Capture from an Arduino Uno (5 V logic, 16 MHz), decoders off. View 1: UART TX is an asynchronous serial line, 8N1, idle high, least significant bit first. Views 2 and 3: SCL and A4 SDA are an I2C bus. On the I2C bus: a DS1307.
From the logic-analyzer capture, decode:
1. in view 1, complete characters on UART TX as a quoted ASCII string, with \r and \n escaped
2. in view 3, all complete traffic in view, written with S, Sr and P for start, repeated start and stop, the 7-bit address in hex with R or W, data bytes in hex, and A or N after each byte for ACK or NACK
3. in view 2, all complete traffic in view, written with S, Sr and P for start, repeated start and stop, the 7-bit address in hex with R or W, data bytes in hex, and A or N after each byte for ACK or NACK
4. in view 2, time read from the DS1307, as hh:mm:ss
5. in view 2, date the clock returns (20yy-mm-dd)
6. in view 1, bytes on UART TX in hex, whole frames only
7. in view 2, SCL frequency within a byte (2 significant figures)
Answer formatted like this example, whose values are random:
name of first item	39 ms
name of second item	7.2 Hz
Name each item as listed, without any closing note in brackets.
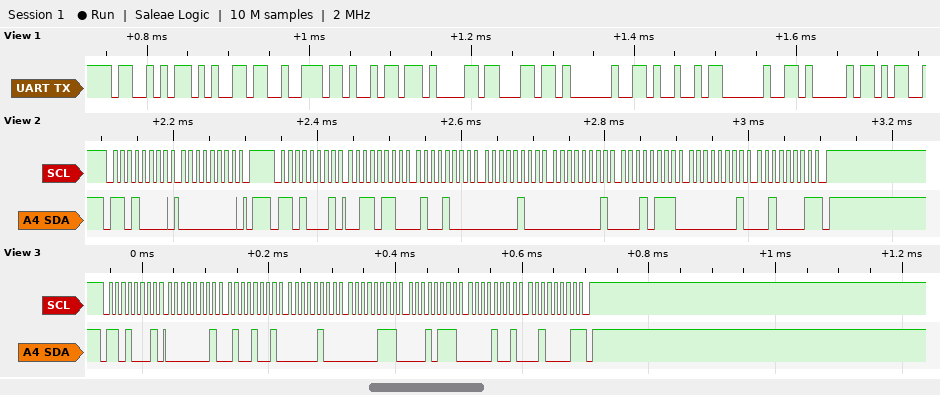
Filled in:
in view 1, complete characters on UART TX as a quoted ASCII string, with \r and \n escaped	"Serial I A"
in view 3, all complete traffic in view, written with S, Sr and P for start, repeated start and stop, the 7-bit address in hex with R or W, data bytes in hex, and A or N after each byte for ACK or NACK	S 68R A 01 A 49 A 04 A 07 A 17 A 09 A 21 N P
in view 2, all complete traffic in view, written with S, Sr and P for start, repeated start and stop, the 7-bit address in hex with R or W, data bytes in hex, and A or N after each byte for ACK or NACK	S 68W A 00 A P S 68R A 36 A 48 A 04 A 01 A 17 A 01 A 21 N P
in view 2, time read from the DS1307, as hh:mm:ss	04:48:36
in view 2, date the clock returns	2021-01-17
in view 1, bytes on UART TX in hex, whole frames only	53 65 72 69 61 6C 20 49 20 41
in view 2, SCL frequency within a byte	100 kHz
